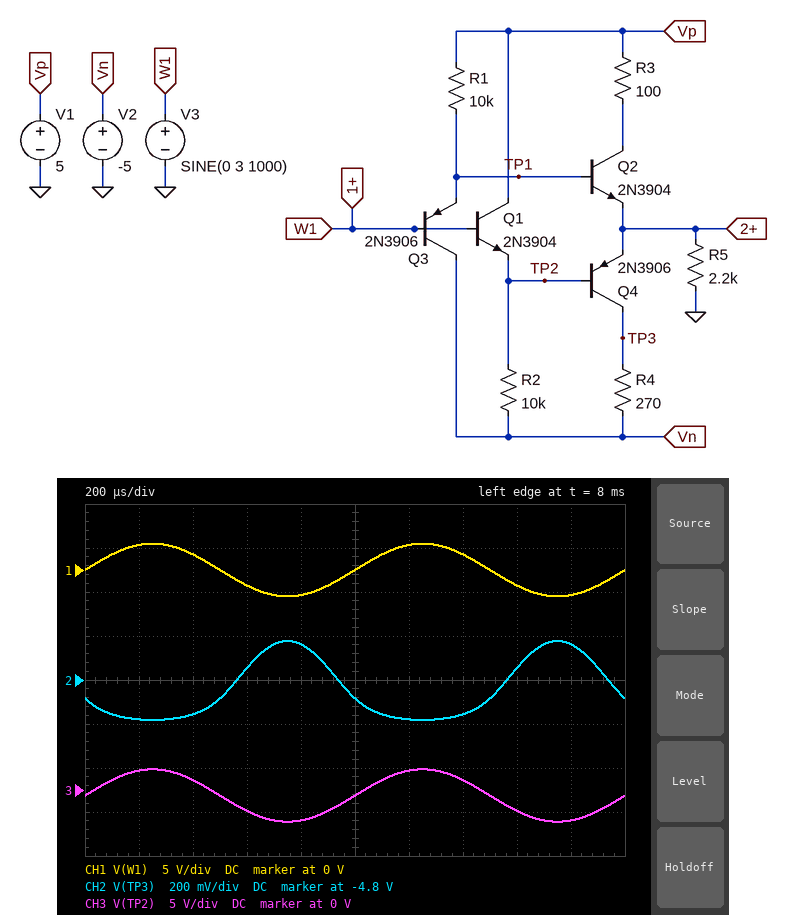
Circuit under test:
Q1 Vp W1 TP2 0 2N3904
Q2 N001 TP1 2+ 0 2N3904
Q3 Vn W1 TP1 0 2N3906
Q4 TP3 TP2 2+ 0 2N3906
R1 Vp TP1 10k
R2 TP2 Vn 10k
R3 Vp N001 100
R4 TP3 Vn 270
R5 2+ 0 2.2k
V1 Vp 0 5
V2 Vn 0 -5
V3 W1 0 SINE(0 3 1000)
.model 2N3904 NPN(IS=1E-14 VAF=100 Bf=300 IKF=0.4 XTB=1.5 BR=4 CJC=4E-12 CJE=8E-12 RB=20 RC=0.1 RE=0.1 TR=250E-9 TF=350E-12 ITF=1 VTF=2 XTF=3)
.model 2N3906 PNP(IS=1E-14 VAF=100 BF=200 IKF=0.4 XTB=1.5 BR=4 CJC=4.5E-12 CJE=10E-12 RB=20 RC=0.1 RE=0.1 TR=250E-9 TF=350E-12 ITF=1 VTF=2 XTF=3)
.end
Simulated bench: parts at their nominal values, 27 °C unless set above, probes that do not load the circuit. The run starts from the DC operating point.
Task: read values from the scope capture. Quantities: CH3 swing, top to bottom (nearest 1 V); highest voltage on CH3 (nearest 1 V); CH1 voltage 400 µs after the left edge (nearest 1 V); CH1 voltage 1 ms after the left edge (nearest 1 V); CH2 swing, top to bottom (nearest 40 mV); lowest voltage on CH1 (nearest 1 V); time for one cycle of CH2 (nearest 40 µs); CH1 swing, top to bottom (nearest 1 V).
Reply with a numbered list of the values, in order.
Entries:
1. 6 V
2. 2 V
3. 2 V
4. 0 V
5. 360 mV
6. -3 V
7. 1.00 ms
8. 6 V
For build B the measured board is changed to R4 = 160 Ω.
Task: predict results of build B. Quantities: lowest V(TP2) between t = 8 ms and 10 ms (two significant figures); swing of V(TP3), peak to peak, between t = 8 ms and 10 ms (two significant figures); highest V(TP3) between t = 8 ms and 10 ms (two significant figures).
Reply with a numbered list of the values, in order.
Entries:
1. -3.6 V
2. 210 mV
3. -4.8 V
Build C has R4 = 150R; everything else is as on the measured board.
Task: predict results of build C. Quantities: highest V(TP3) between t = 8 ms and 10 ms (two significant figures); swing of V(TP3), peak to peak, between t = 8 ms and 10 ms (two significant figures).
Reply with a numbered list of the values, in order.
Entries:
1. -4.8 V
2. 200 mV
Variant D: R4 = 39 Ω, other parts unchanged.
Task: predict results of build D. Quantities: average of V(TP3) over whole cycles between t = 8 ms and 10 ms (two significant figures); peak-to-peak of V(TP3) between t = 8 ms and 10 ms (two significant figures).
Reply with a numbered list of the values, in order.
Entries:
1. -5.0 V
2. 52 mV
